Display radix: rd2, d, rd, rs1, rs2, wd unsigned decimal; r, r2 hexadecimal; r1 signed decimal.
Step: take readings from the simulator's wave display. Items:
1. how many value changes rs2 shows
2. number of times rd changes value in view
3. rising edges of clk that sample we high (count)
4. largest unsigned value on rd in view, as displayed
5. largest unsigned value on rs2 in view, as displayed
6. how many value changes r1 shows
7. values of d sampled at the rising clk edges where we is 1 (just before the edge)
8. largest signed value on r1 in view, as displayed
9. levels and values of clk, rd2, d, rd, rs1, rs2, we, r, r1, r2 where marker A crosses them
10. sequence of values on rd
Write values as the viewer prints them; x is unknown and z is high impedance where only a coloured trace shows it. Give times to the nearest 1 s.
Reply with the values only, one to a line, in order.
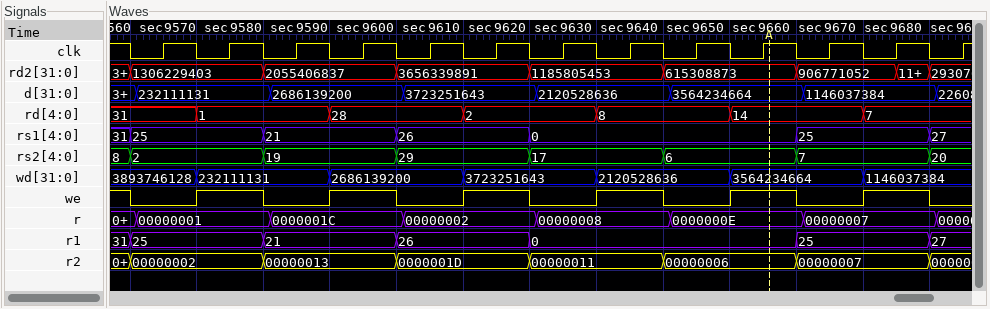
7
6
6
31
29
6
232111131, 2686139200, 3723251643, 2120528636, 3564234664, 1146037384
31
clk=1, rd2=615308873, d=3564234664, rd=14, rs1=0, rs2=6, we=1, r=0000000E, r1=0, r2=00000006
31, 1, 28, 2, 8, 14, 7
